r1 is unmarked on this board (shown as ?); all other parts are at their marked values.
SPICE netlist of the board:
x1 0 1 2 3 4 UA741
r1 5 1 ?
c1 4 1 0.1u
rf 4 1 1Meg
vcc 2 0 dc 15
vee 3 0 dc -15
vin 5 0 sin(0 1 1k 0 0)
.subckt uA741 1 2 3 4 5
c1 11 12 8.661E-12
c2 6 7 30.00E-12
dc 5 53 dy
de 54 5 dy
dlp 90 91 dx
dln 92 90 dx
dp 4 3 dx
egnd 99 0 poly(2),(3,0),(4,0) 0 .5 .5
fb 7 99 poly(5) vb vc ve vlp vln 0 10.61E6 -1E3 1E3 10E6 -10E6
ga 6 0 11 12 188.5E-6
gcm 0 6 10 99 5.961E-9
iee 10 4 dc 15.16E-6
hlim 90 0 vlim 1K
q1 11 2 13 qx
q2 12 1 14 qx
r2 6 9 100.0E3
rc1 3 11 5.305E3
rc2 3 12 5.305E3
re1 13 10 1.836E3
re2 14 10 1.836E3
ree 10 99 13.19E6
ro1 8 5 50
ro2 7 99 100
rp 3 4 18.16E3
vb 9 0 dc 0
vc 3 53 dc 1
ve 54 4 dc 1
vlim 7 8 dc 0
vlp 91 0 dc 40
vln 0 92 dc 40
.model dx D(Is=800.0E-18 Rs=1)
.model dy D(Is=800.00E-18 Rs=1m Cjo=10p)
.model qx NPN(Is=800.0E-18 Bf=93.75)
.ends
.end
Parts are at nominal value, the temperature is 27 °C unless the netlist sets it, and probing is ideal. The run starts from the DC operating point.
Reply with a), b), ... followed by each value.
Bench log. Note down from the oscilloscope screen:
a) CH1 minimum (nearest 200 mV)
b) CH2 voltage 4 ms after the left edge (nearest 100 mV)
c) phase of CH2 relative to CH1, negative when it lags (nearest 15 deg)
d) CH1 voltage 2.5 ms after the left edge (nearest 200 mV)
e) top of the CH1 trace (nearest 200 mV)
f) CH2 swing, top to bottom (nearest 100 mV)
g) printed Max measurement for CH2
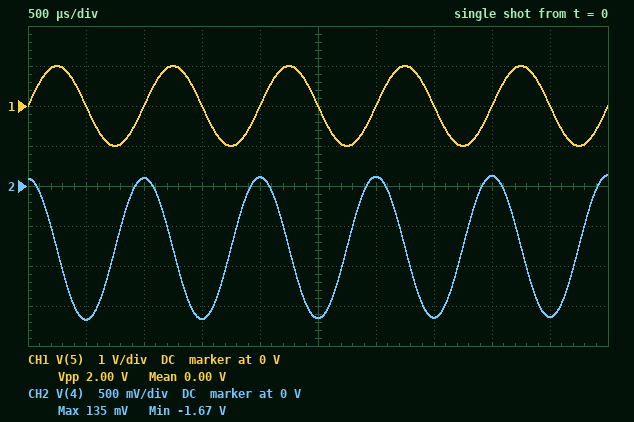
a) -1.0 V
b) 100 mV
c) 90 deg
d) 0 V
e) 1.0 V
f) 1.8 V
g) 135 mV
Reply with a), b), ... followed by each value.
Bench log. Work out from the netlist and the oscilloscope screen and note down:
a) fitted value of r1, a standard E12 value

a) 1.8 kΩ
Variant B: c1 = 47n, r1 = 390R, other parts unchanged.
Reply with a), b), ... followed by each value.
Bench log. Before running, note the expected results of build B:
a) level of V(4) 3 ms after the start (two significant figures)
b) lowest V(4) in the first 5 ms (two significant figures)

a) 2.7 V
b) -15 V
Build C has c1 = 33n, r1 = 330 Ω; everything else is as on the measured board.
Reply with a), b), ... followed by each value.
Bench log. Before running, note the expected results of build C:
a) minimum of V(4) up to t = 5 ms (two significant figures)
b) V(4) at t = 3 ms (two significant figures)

a) -15 V
b) 14 V
